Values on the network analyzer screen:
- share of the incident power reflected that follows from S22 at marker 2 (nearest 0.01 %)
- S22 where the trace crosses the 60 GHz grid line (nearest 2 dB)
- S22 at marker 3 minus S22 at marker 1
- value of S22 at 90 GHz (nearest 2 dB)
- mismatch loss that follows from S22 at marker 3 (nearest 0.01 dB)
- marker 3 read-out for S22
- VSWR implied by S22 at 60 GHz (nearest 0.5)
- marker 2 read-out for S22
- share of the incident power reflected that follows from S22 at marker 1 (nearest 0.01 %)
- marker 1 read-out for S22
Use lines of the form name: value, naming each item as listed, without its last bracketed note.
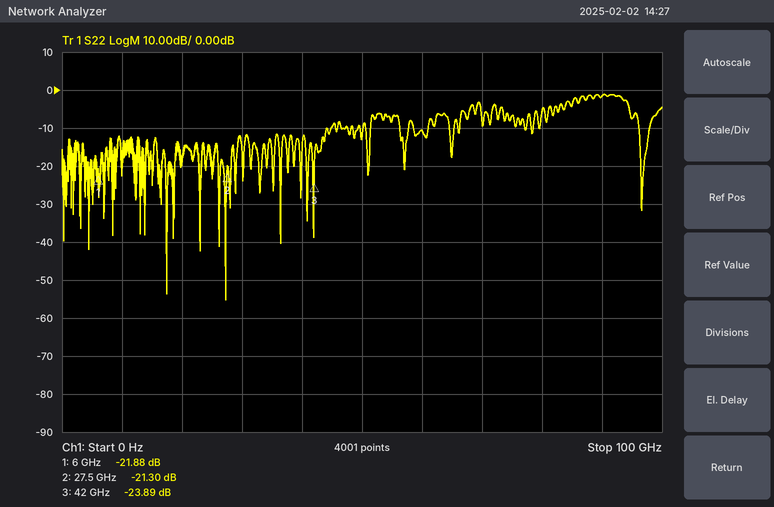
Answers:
share of the incident power reflected that follows from S22 at marker 2: 0.74 %
S22 where the trace crosses the 60 GHz grid line: -10 dB
S22 at marker 3 minus S22 at marker 1: -2.01 dB
value of S22 at 90 GHz: -2 dB
mismatch loss that follows from S22 at marker 3: 0.02 dB
marker 3 read-out for S22: -23.89 dB
VSWR implied by S22 at 60 GHz: 2.0
marker 2 read-out for S22: -21.30 dB
share of the incident power reflected that follows from S22 at marker 1: 0.65 %
marker 1 read-out for S22: -21.88 dB
